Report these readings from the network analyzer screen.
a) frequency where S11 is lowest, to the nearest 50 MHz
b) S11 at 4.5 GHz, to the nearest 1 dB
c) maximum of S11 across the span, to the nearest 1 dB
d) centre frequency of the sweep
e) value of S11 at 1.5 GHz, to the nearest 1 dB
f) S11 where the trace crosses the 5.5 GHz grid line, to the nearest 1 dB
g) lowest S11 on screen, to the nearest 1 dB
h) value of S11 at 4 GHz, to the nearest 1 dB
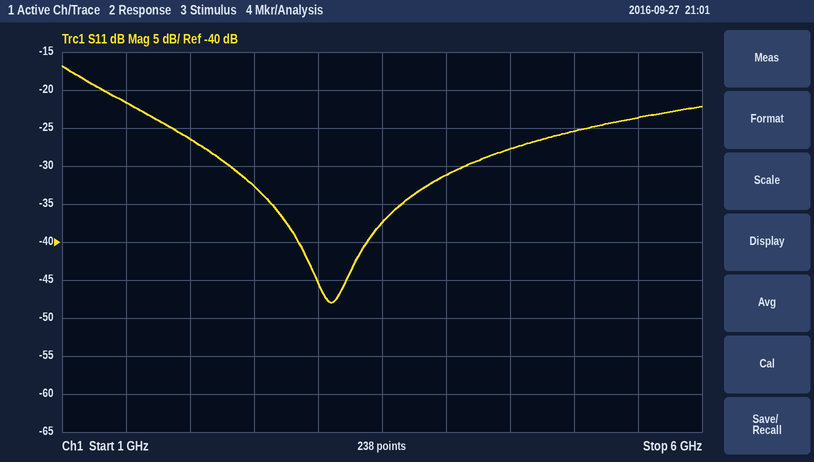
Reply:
3.10 GHz
-28 dB
-17 dB
3.5 GHz
-22 dB
-24 dB
-48 dB
-31 dB
